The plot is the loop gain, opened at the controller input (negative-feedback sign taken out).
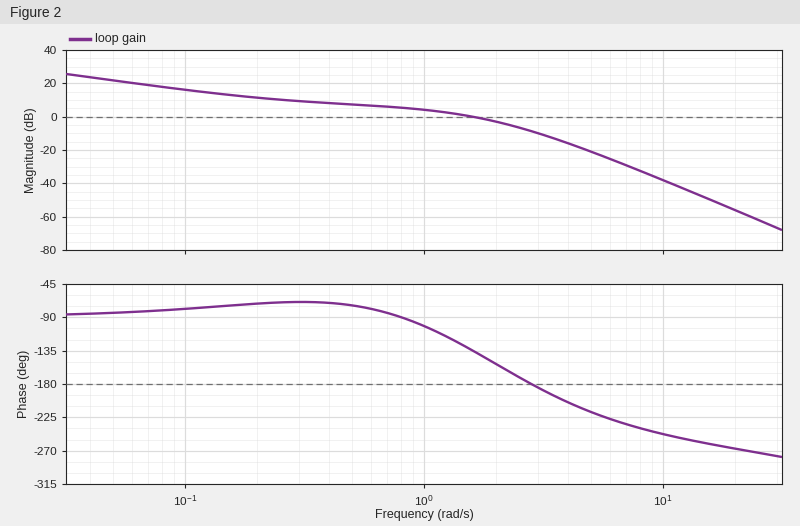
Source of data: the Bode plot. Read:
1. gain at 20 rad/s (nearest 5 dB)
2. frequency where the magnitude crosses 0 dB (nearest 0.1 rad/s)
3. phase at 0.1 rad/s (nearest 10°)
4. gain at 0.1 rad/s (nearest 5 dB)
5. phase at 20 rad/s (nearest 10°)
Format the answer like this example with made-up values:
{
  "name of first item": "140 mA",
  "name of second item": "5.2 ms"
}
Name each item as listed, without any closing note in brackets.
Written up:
{
  "gain at 20 rad/s": "-55 dB",
  "frequency where the magnitude crosses 0 dB": "1.6 rad/s",
  "phase at 0.1 rad/s": "-80°",
  "gain at 0.1 rad/s": "15 dB",
  "phase at 20 rad/s": "-270°"
}
